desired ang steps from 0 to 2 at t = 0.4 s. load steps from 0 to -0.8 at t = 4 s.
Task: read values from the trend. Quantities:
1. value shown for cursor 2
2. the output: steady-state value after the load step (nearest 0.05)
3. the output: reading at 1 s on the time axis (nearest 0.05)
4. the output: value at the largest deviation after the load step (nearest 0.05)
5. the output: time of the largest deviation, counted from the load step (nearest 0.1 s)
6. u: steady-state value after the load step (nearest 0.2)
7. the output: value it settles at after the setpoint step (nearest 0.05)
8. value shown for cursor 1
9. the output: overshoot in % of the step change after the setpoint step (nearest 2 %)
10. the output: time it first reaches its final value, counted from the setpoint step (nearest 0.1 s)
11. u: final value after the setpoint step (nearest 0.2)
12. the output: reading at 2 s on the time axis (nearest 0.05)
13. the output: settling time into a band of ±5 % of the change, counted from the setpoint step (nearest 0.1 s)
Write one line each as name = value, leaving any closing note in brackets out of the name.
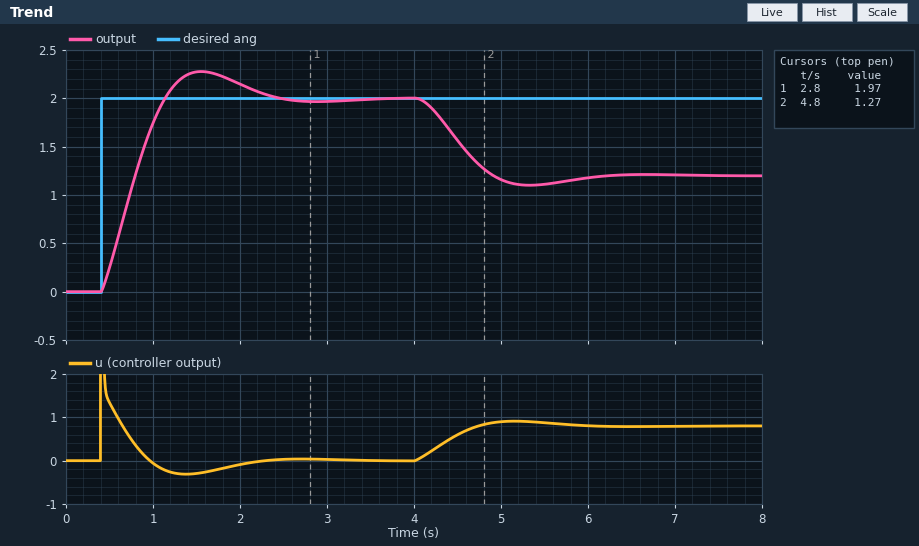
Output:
value shown for cursor 2 = 1.27
the output: steady-state value after the load step = 1.20
the output: reading at 1 s on the time axis = 1.75
the output: value at the largest deviation after the load step = 1.10
the output: time of the largest deviation, counted from the load step = 1.3 s
u: steady-state value after the load step = 0.8
the output: value it settles at after the setpoint step = 2.00
value shown for cursor 1 = 1.97
the output: overshoot in % of the step change after the setpoint step = 14 %
the output: time it first reaches its final value, counted from the setpoint step = 0.7 s
u: final value after the setpoint step = 0.0
the output: reading at 2 s on the time axis = 2.15
the output: settling time into a band of ±5 % of the change, counted from the setpoint step = 1.7 s
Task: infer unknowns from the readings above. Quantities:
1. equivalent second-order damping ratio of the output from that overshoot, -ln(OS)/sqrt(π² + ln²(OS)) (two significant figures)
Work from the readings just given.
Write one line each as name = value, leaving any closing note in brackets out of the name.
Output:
equivalent second-order damping ratio of the output from that overshoot, -ln(OS)/sqrt(π² + ln²(OS)) = 0.53
